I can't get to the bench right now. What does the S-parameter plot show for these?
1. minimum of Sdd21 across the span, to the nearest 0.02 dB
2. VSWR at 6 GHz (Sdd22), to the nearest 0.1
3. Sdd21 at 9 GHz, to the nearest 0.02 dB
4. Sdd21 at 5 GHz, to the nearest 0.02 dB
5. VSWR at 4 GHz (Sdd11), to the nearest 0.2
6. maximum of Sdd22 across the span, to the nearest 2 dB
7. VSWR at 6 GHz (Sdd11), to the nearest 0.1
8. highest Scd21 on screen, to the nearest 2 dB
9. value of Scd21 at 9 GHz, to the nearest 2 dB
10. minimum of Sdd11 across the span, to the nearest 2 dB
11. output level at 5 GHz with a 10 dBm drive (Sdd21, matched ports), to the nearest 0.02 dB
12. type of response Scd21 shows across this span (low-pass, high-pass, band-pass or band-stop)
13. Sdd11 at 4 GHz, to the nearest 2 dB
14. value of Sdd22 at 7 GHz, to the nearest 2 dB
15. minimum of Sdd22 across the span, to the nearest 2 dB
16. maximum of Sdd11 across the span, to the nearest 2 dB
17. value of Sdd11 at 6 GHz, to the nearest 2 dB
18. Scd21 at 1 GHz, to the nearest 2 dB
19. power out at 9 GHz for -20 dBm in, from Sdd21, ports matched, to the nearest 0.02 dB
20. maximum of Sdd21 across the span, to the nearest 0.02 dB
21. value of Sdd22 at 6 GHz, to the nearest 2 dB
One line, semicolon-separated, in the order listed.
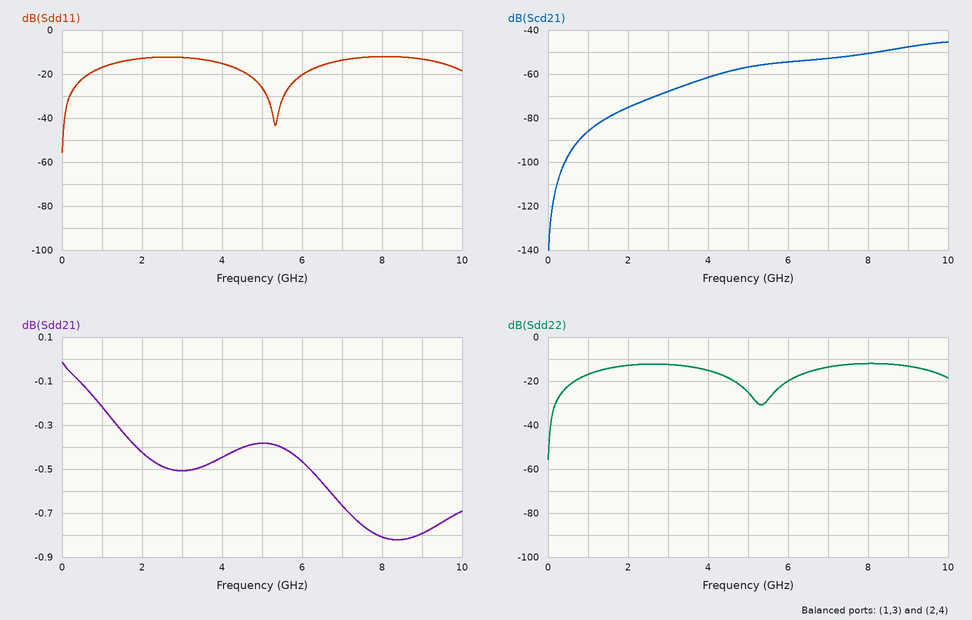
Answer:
-0.82 dB; 1.2; -0.80 dB; -0.38 dB; 1.4; -12 dB; 1.2; -46 dB; -48 dB; -56 dB; 9.62 dBm; high-pass; -16 dB; -14 dB; -56 dB; -12 dB; -20 dB; -86 dB; -20.80 dBm; -0.02 dB; -20 dB
